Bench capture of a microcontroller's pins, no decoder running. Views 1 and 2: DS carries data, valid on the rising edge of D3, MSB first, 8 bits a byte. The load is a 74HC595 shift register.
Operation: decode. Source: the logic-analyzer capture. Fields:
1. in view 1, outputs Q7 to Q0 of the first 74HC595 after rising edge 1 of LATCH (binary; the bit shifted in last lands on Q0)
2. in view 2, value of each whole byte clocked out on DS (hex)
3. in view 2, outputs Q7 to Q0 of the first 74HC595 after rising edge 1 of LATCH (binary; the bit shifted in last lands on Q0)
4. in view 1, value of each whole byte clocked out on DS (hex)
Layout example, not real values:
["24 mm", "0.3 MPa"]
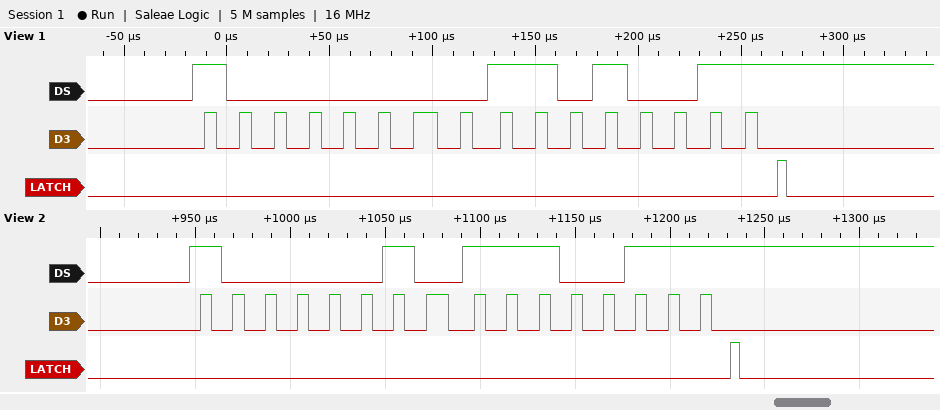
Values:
["11010011", "0x82 0xE7", "11100111", "0x80 0xD3"]
